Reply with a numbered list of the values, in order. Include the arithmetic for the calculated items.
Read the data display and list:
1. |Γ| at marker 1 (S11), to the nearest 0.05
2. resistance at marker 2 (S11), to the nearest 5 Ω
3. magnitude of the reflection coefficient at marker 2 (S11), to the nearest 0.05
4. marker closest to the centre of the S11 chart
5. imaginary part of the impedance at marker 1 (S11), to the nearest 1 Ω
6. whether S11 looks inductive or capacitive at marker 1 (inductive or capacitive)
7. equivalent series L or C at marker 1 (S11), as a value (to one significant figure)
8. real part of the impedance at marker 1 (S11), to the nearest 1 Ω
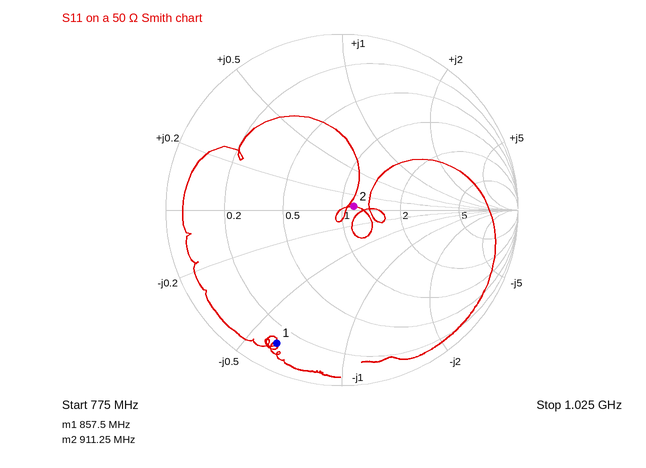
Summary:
1. 0.85
2. 55 Ω
3. 0.05
4. marker 2
5. -31 Ω
6. capacitive
7. C = 1/(2π × 857.5 MHz × 31 Ω) ≈ 6 pF
8. 6 Ω
